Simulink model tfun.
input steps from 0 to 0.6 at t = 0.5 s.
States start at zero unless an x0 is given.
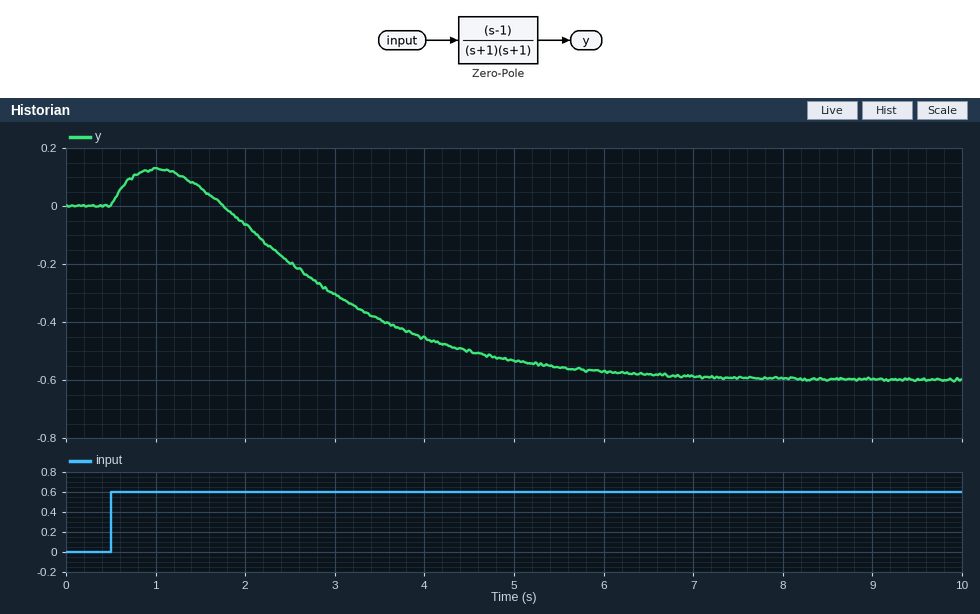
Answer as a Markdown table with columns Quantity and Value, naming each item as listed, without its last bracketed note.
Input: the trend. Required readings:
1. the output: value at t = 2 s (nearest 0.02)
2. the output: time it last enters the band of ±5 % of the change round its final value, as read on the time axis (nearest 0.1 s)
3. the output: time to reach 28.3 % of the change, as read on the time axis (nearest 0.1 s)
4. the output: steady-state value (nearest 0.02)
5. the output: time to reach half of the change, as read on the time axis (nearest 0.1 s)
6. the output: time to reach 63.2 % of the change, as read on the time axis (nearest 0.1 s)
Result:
| Quantity | Value |
|---|---|
| the output: value at t = 2 s | -0.06 |
| the output: time it last enters the band of ±5 % of the change round its final value, as read on the time axis | 6.0 s |
| the output: time to reach 28.3 % of the change, as read on the time axis | 2.4 s |
| the output: steady-state value | -0.60 |
| the output: time to reach half of the change, as read on the time axis | 3.0 s |
| the output: time to reach 63.2 % of the change, as read on the time axis | 3.4 s |
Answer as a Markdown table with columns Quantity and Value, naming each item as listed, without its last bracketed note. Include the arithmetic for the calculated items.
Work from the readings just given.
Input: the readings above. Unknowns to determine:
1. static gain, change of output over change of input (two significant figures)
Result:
| Quantity | Value |
|---|---|
| static gain, change of output over change of input | (-0.6 - 0) / (0.6 - 0) = -1.0 |
